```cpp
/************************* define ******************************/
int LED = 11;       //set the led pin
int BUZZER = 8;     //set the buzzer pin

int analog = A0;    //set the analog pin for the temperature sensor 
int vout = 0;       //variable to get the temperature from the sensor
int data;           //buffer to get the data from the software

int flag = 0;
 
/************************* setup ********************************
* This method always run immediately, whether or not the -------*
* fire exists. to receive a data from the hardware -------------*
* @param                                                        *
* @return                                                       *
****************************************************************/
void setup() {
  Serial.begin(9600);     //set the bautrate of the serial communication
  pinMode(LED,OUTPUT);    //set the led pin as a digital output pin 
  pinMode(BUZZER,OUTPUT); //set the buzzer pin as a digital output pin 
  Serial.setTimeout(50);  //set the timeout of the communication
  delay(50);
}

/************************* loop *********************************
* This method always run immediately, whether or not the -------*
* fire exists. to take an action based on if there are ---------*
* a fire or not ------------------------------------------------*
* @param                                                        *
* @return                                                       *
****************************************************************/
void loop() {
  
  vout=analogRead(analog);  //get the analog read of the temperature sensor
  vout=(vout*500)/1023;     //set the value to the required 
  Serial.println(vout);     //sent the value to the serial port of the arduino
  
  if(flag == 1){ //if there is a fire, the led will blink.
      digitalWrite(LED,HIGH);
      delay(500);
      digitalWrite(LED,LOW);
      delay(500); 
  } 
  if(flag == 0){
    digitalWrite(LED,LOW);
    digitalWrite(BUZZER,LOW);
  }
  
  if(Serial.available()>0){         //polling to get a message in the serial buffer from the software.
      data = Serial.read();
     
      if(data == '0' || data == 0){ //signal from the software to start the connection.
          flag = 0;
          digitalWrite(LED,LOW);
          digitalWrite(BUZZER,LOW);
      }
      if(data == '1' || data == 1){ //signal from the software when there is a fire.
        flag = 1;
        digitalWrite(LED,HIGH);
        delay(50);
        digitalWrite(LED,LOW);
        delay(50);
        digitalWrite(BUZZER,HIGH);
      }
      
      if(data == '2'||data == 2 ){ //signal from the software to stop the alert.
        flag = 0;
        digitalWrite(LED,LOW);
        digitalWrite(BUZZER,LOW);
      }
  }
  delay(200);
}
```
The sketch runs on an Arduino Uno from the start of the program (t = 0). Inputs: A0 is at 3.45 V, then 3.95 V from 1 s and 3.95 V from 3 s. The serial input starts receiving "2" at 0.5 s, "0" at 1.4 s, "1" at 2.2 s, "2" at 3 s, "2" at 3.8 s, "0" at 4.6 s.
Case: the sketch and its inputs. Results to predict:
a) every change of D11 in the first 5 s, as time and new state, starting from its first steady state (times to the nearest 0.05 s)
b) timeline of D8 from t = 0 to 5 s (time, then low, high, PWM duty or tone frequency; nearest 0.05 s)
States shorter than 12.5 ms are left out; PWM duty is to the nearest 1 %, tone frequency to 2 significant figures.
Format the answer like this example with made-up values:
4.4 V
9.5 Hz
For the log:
0 s low; 2.25 s high; 2.3 s low; 2.55 s high; 3.05 s low
0 s low; 2.35 s high; 3.55 s low
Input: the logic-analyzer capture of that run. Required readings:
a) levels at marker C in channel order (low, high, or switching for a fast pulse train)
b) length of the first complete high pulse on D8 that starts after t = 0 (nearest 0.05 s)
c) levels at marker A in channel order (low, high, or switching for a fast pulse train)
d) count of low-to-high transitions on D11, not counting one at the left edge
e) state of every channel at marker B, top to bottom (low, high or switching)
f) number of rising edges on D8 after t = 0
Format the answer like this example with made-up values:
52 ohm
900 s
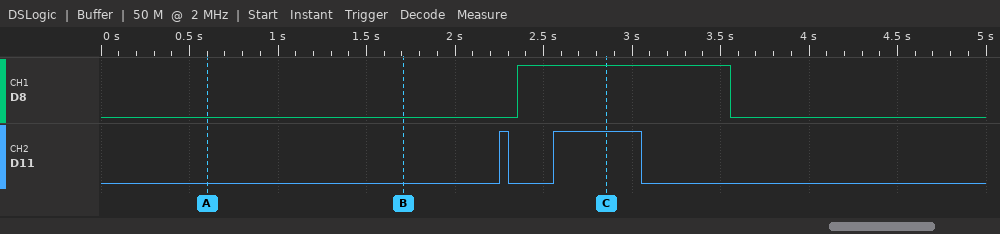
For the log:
D8 high, D11 high
1.20 s
D8 low, D11 low
2
D8 low, D11 low
1
